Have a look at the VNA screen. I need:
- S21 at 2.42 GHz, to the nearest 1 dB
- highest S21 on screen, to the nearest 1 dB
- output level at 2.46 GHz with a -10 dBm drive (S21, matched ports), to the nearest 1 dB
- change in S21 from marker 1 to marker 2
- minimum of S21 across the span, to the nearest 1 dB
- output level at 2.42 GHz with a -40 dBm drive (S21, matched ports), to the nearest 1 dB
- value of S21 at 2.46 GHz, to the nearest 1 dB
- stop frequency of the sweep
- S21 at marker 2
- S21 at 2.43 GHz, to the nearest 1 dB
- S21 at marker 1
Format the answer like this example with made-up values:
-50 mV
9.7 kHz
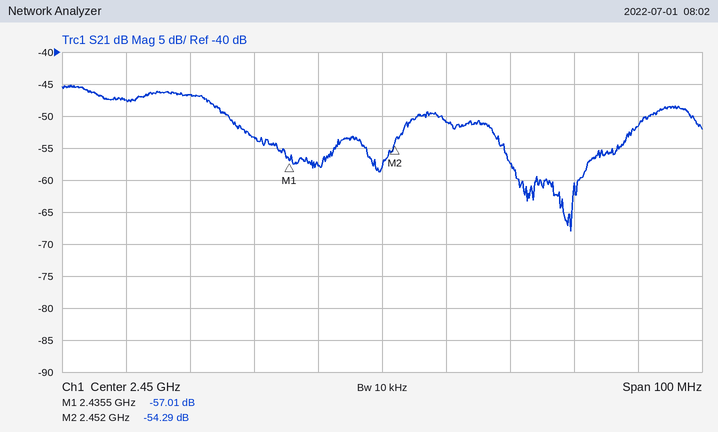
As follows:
-47 dB
-45 dB
-61 dBm
2.72 dB
-68 dB
-87 dBm
-51 dB
2.5 GHz
-54.29 dB
-53 dB
-57.01 dB
